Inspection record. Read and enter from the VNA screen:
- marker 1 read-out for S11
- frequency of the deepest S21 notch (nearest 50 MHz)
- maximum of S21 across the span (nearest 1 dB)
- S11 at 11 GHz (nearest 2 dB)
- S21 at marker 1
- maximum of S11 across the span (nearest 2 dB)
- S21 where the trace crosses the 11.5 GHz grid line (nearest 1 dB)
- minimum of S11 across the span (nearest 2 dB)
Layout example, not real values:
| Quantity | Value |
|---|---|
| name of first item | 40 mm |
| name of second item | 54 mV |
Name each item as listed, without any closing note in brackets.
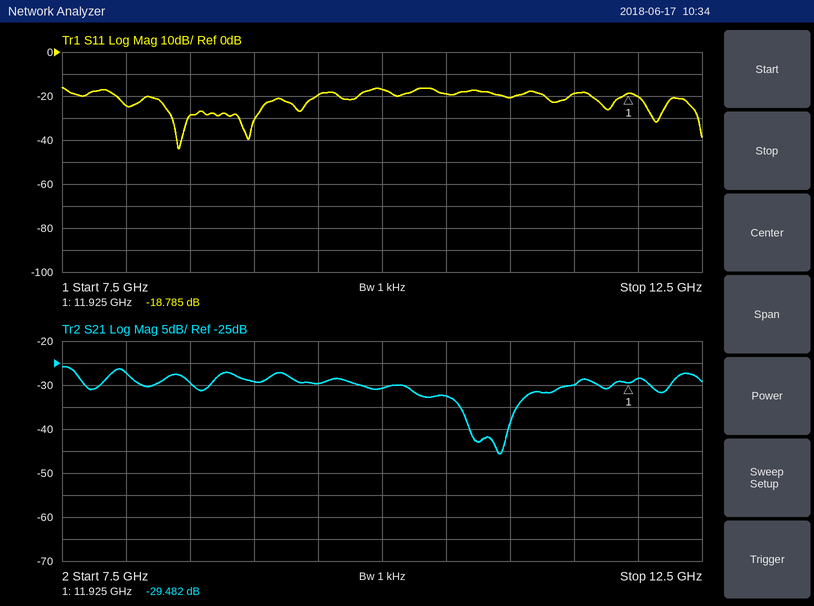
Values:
| Quantity | Value |
|---|---|
| marker 1 read-out for S11 | -18.785 dB |
| frequency of the deepest S21 notch | 10.90 GHz |
| maximum of S21 across the span | -26 dB |
| S11 at 11 GHz | -20 dB |
| S21 at marker 1 | -29.482 dB |
| maximum of S11 across the span | -16 dB |
| S21 where the trace crosses the 11.5 GHz grid line | -30 dB |
| minimum of S11 across the span | -44 dB |
